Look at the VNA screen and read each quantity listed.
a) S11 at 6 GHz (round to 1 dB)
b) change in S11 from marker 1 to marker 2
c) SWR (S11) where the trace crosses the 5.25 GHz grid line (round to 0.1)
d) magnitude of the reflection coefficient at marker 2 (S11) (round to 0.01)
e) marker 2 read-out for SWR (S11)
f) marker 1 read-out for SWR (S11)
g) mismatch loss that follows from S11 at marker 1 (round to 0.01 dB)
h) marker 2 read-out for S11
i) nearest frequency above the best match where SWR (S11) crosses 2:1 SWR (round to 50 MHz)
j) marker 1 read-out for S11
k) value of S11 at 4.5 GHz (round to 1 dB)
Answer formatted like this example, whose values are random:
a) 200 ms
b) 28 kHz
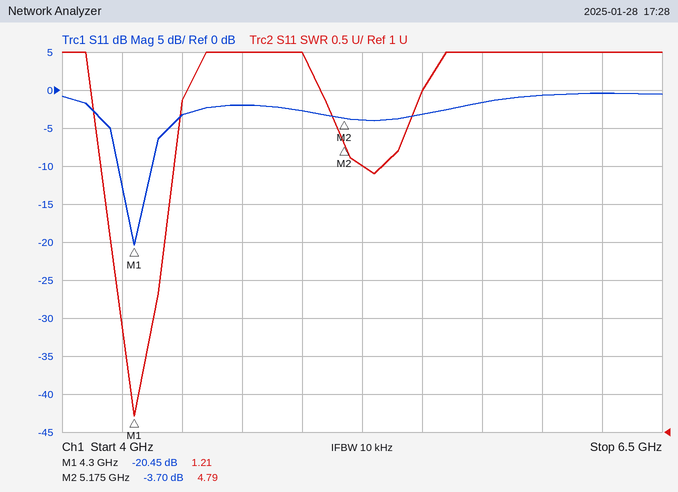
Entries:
a) -1 dB
b) 16.75 dB
c) 4.5
d) 0.65
e) 4.79
f) 1.21
g) 0.04 dB
h) -3.70 dB
i) 4.35 GHz
j) -20.45 dB
k) -3 dB
